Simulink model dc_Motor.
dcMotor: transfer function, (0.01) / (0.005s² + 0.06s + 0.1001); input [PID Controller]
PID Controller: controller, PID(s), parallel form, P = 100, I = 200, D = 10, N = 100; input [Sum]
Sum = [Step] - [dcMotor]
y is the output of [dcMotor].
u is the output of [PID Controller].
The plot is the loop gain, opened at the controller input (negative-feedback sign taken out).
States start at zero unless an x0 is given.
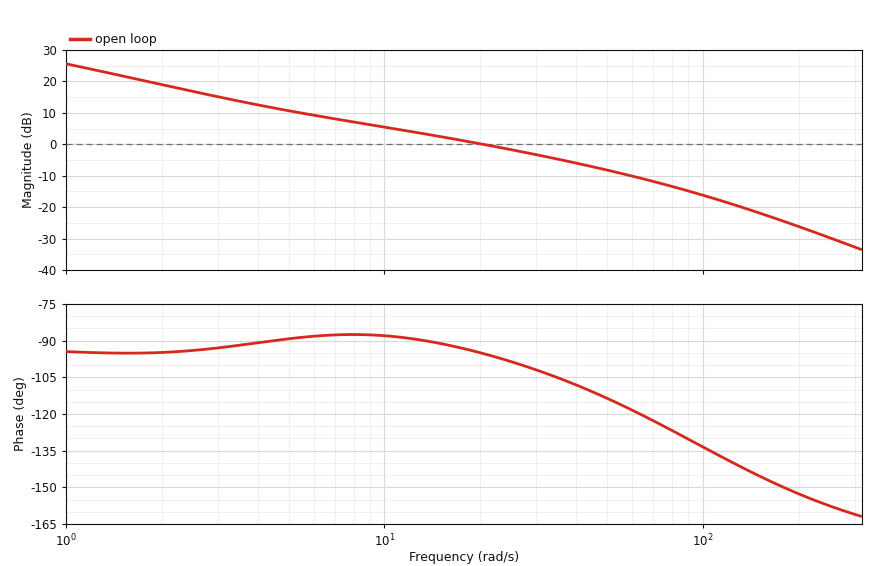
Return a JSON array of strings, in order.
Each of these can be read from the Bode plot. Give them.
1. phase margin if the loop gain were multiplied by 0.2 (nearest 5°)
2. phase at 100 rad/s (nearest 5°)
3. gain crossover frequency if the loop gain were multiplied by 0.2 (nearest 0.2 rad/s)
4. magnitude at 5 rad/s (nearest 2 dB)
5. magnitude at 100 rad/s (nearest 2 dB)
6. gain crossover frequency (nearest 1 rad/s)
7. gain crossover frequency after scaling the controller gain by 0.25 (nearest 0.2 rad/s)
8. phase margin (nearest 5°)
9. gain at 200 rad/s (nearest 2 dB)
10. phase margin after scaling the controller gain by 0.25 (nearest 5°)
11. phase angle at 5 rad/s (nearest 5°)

["90°", "-135°", "3.4 rad/s", "10 dB", "-16 dB", "20 rad/s", "4.2 rad/s", "85°", "-26 dB", "90°", "-90°"]
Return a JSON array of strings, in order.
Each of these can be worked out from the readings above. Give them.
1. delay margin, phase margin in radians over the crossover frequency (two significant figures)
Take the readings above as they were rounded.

["0.074 s"]
